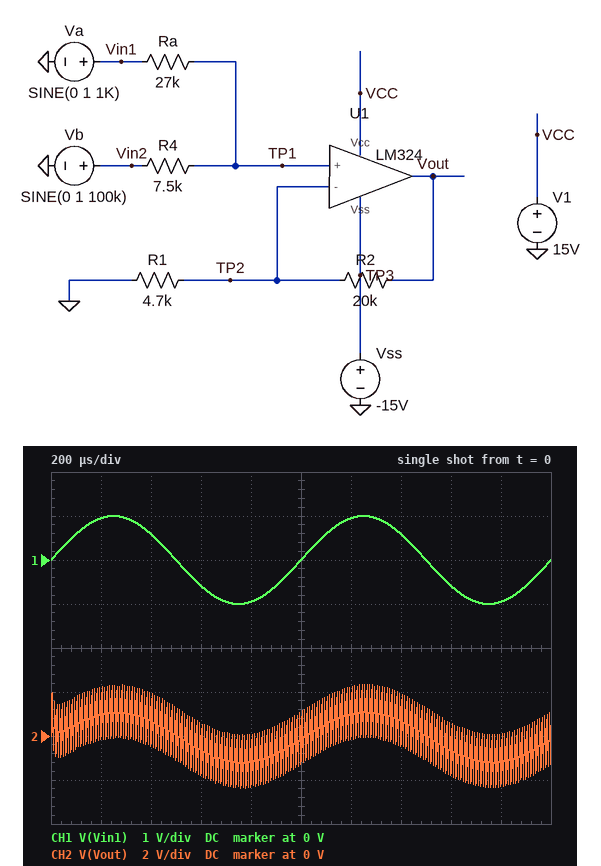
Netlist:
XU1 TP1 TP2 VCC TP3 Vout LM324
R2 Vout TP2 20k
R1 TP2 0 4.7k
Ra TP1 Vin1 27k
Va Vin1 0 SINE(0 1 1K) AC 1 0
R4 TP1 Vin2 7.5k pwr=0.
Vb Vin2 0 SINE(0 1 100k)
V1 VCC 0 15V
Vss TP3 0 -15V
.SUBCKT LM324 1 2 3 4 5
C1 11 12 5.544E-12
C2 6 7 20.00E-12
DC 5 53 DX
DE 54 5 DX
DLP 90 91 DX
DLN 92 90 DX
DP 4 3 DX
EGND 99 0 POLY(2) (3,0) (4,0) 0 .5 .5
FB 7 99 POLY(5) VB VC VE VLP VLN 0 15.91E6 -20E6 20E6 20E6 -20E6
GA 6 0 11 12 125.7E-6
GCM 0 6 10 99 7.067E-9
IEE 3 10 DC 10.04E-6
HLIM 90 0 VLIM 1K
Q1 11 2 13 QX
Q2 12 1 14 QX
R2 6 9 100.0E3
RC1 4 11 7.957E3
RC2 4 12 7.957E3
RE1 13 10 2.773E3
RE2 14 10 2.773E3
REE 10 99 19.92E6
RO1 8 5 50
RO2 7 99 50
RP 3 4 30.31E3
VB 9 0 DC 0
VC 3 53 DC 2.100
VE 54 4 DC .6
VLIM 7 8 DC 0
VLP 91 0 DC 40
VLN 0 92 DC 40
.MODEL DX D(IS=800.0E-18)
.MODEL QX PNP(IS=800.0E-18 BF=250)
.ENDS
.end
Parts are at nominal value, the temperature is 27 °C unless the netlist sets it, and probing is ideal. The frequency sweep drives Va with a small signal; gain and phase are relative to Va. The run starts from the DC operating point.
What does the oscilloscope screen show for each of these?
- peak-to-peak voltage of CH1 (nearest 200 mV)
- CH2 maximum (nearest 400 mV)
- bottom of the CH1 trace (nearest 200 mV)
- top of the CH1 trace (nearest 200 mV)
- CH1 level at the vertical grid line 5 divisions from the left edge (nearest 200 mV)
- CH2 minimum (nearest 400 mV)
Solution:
2.0 V
2.4 V
-1.0 V
1.0 V
0 V
-2.4 V
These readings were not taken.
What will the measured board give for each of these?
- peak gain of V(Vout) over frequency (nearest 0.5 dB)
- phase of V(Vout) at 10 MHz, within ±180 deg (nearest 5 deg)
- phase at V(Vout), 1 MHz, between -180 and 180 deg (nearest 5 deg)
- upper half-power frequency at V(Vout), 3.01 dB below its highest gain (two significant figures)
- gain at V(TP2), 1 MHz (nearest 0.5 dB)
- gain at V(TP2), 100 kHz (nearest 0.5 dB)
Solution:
1.0 dB
-170 deg
-110 deg
210 kHz
-28.5 dB
-14.0 dB
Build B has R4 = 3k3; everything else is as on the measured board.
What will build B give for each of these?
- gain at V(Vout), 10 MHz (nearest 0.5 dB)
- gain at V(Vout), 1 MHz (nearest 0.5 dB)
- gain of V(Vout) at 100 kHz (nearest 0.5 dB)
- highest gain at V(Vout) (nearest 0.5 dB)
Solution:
-54.5 dB
-20.0 dB
-5.5 dB
-5.0 dB
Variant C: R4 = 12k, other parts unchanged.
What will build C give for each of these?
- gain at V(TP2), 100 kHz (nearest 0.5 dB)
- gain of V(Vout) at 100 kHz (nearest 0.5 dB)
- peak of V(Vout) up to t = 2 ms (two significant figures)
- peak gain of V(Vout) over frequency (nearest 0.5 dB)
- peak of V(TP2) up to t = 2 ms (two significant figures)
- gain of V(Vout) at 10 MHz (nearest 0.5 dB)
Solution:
-11.0 dB
3.5 dB
2.8 V
4.0 dB
530 mV
-45.5 dB
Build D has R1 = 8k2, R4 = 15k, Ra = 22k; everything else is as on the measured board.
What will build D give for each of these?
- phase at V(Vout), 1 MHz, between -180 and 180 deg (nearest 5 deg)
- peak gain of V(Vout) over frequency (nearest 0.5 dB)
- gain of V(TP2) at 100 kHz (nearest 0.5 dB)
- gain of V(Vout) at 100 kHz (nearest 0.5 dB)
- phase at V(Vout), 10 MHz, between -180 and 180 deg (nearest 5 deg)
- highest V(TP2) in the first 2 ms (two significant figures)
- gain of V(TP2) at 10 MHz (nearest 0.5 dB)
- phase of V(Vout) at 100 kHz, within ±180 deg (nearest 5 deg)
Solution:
-105 deg
3.0 dB
-8.0 dB
2.5 dB
-170 deg
740 mV
-56.5 dB
-20 deg
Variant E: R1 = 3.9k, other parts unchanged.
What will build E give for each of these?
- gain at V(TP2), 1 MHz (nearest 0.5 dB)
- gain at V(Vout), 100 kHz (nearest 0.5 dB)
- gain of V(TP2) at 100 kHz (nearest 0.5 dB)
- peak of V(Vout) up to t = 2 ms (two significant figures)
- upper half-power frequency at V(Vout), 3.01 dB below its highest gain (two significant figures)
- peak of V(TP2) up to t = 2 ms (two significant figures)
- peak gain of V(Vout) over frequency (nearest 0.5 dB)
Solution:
-29.5 dB
1.5 dB
-14.5 dB
2.5 V
180 kHz
410 mV
2.5 dB
